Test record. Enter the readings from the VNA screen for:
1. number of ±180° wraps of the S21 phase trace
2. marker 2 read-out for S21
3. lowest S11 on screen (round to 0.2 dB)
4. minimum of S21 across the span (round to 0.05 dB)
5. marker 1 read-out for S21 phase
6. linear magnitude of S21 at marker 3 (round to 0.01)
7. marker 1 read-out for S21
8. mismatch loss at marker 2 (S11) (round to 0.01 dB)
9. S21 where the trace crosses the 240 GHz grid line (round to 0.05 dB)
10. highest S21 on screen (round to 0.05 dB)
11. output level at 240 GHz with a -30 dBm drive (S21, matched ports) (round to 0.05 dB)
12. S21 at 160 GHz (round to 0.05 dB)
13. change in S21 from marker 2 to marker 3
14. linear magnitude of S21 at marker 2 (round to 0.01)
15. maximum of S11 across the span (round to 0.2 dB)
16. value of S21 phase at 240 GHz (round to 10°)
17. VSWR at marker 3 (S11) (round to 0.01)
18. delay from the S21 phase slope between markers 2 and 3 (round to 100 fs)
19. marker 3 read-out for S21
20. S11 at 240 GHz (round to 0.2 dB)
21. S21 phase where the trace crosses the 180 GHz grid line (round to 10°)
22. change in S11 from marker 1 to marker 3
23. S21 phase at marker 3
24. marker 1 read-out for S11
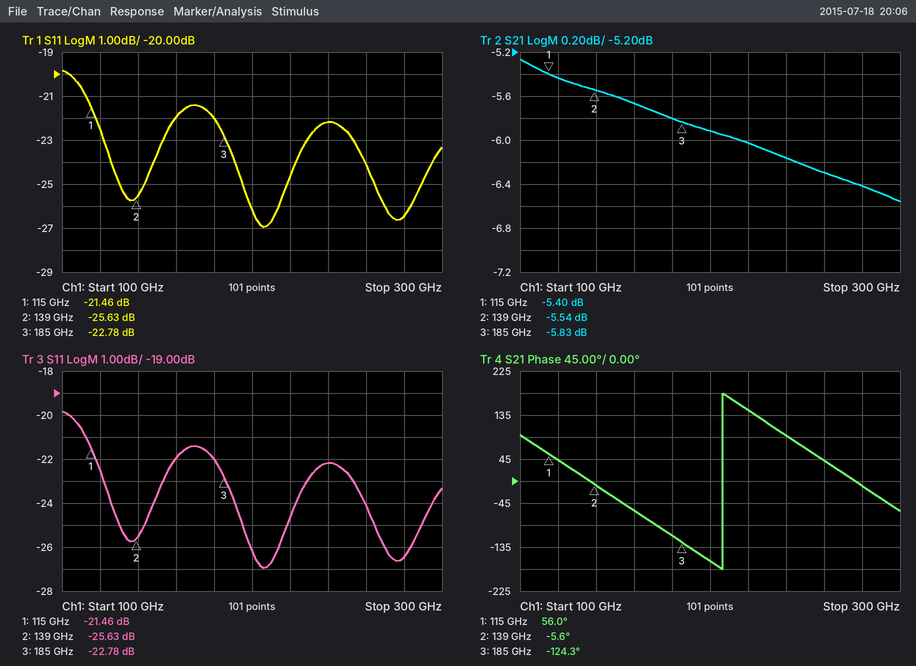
1
-5.54 dB
-27.0 dB
-6.55 dB
56.0°
0.51
-5.40 dB
0.01 dB
-6.15 dB
-5.25 dB
-36.15 dBm
-5.65 dB
-0.29 dB
0.53
-19.8 dB
90°
1.16
7.2 ps
-5.83 dB
-22.2 dB
-110°
-1.32 dB
-124.3°
-21.46 dB
